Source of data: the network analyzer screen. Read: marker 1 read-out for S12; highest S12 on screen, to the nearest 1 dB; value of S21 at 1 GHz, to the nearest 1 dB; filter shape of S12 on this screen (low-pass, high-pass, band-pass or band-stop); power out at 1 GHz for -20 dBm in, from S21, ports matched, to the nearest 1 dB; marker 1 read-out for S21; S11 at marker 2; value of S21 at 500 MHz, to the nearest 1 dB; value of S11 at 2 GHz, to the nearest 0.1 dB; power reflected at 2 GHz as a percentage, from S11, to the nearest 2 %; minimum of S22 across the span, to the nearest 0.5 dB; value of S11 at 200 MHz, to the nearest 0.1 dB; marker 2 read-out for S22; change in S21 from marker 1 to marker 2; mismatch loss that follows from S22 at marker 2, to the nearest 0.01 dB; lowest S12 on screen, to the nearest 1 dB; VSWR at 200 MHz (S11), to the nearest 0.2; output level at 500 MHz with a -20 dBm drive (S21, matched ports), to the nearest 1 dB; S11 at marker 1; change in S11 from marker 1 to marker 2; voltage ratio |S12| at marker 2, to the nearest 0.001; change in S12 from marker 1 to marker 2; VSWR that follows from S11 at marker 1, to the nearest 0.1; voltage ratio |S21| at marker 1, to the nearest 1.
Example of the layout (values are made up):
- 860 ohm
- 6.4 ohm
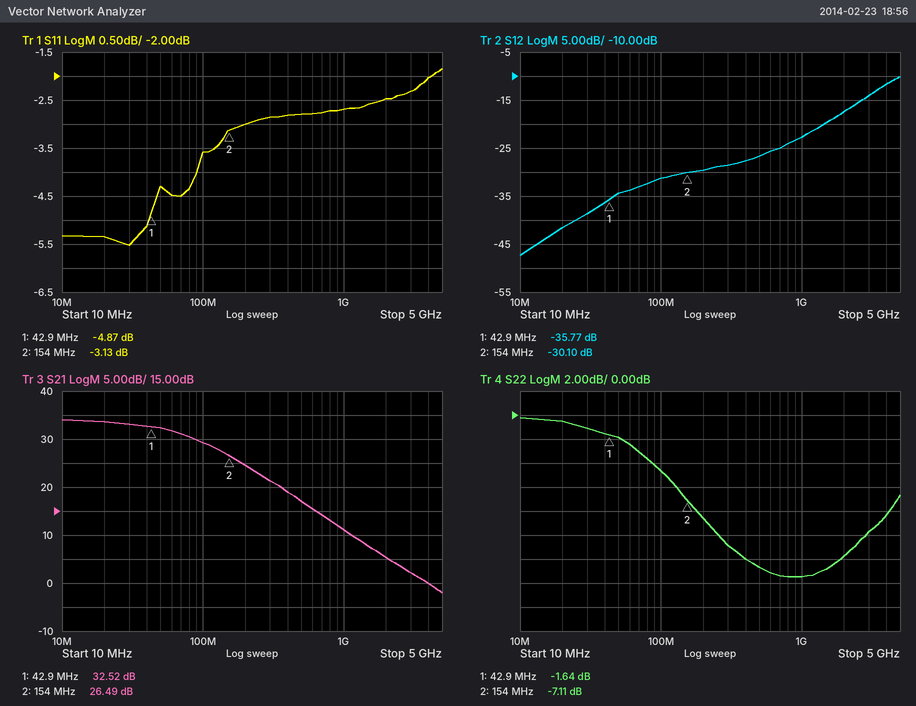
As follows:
- -35.77 dB
- -10 dB
- 11 dB
- high-pass
- -9 dBm
- 32.52 dB
- -3.13 dB
- 17 dB
- -2.5 dB
- 56 %
- -13.5 dB
- -3.0 dB
- -7.11 dB
- -6.03 dB
- 0.94 dB
- -47 dB
- 5.8
- -3 dBm
- -4.87 dB
- 1.74 dB
- 0.031
- 5.67 dB
- 3.7
- 42
